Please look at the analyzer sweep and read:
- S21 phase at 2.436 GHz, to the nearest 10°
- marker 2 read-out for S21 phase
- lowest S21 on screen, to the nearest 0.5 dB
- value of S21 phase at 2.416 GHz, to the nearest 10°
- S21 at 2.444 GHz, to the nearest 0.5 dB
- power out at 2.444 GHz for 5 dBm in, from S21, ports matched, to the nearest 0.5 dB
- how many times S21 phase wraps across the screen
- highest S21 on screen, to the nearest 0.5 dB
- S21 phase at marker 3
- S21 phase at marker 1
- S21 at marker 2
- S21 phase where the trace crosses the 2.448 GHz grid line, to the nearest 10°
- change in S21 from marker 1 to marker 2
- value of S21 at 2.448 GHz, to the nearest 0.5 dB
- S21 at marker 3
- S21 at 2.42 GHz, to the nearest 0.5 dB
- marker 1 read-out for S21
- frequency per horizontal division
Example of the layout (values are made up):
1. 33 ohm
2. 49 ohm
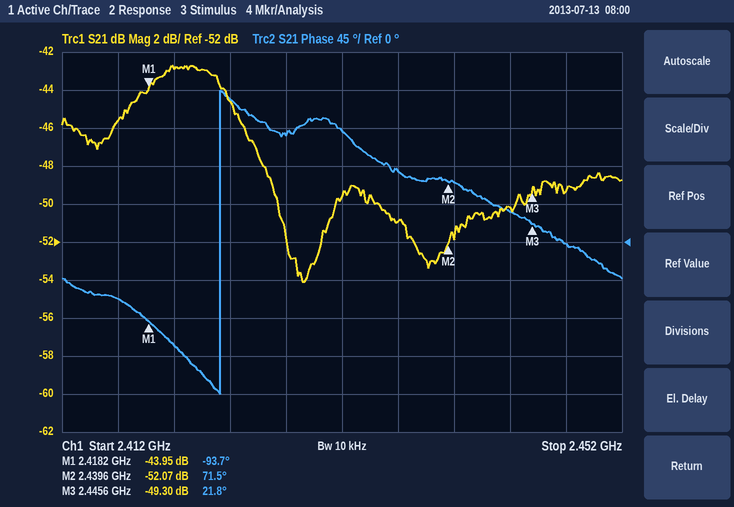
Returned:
1. 80°
2. 71.5°
3. -54.0 dB
4. -70°
5. -50.0 dB
6. -45.0 dBm
7. 1
8. -42.5 dB
9. 21.8°
10. -93.7°
11. -52.07 dB
12. 0°
13. -8.12 dB
14. -49.5 dB
15. -49.30 dB
16. -43.0 dB
17. -43.95 dB
18. 4 MHz
